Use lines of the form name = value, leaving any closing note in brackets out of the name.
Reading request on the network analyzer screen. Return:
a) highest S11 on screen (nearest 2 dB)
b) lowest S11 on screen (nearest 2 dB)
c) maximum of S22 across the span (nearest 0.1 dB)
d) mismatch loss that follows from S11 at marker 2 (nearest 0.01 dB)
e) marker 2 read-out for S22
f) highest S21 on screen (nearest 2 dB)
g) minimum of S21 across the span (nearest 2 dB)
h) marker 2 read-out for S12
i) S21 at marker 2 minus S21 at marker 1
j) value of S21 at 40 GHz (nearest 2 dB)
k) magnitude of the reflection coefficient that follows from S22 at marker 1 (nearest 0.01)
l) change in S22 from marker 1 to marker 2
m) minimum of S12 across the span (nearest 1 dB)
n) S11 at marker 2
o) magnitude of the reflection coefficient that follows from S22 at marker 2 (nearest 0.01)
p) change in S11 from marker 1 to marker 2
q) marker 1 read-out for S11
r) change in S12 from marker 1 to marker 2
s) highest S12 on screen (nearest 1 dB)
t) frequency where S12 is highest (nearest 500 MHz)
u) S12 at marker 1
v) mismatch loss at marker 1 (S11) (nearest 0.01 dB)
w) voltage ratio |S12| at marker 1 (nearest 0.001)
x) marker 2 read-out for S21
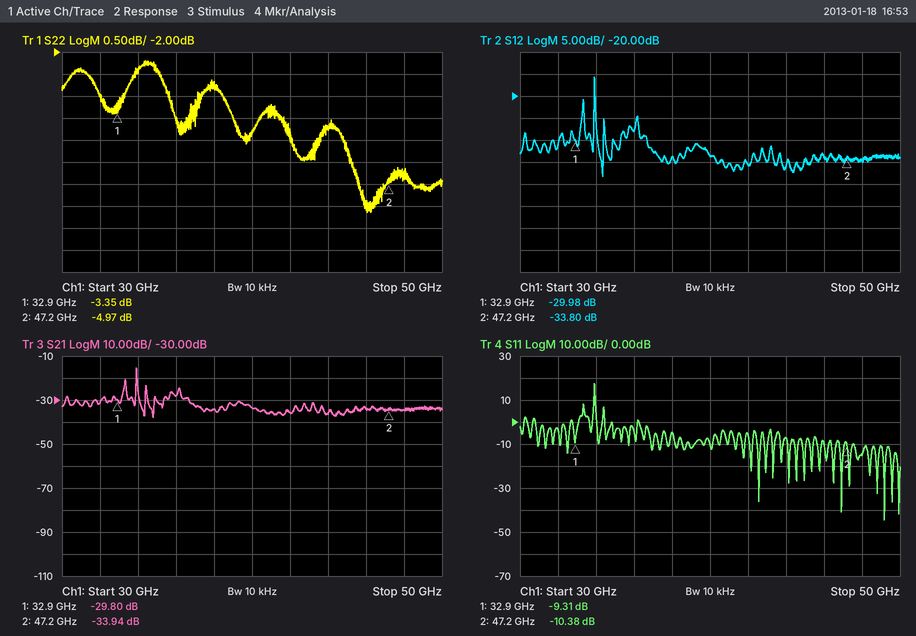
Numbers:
highest S11 on screen = 18 dB
lowest S11 on screen = -44 dB
maximum of S22 across the span = -2.2 dB
mismatch loss that follows from S11 at marker 2 = 0.42 dB
marker 2 read-out for S22 = -4.97 dB
highest S21 on screen = -16 dB
minimum of S21 across the span = -38 dB
marker 2 read-out for S12 = -33.80 dB
S21 at marker 2 minus S21 at marker 1 = -4.14 dB
value of S21 at 40 GHz = -34 dB
magnitude of the reflection coefficient that follows from S22 at marker 1 = 0.68
change in S22 from marker 1 to marker 2 = -1.62 dB
minimum of S12 across the span = -38 dB
S11 at marker 2 = -10.38 dB
magnitude of the reflection coefficient that follows from S22 at marker 2 = 0.56
change in S11 from marker 1 to marker 2 = -1.07 dB
marker 1 read-out for S11 = -9.31 dB
change in S12 from marker 1 to marker 2 = -3.82 dB
highest S12 on screen = -16 dB
frequency where S12 is highest = 34.0 GHz
S12 at marker 1 = -29.98 dB
mismatch loss at marker 1 (S11) = 0.54 dB
voltage ratio |S12| at marker 1 = 0.032
marker 2 read-out for S21 = -33.94 dB
